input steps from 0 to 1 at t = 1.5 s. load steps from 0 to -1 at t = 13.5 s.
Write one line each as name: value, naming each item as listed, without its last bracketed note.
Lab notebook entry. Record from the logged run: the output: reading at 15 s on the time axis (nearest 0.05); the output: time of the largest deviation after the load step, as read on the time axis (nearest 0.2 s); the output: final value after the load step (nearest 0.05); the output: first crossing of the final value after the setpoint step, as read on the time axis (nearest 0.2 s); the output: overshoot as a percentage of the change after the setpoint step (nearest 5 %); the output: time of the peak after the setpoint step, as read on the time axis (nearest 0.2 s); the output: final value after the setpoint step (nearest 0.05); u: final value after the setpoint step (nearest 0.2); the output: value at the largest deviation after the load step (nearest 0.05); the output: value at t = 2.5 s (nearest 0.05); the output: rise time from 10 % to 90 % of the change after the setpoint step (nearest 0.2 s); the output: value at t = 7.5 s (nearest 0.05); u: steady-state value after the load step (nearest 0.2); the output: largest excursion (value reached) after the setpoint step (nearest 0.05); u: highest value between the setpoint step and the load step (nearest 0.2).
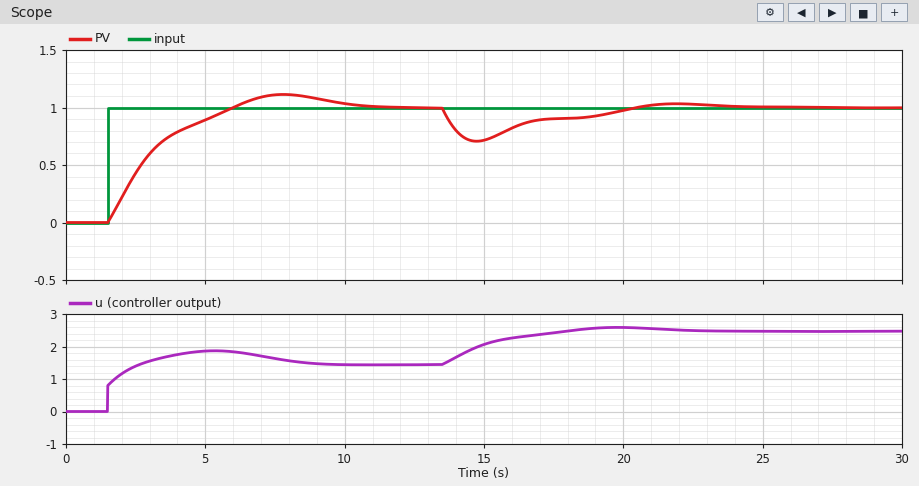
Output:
the output: reading at 15 s on the time axis: 0.70
the output: time of the largest deviation after the load step, as read on the time axis: 14.8 s
the output: final value after the load step: 1.00
the output: first crossing of the final value after the setpoint step, as read on the time axis: 6.0 s
the output: overshoot as a percentage of the change after the setpoint step: 10 %
the output: time of the peak after the setpoint step, as read on the time axis: 7.8 s
the output: final value after the setpoint step: 1.00
u: final value after the setpoint step: 1.4
the output: value at the largest deviation after the load step: 0.70
the output: value at t = 2.5 s: 0.45
the output: rise time from 10 % to 90 % of the change after the setpoint step: 3.4 s
the output: value at t = 7.5 s: 1.10
u: steady-state value after the load step: 2.4
the output: largest excursion (value reached) after the setpoint step: 1.10
u: highest value between the setpoint step and the load step: 1.8
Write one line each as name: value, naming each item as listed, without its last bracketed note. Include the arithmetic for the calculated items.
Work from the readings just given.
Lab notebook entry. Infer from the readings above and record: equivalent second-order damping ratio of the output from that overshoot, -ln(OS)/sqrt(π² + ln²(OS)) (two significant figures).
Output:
equivalent second-order damping ratio of the output from that overshoot, -ln(OS)/sqrt(π² + ln²(OS)): ln(0.1) = -2.303; 2.303 / sqrt(9.870 + 5.302) = 0.59
